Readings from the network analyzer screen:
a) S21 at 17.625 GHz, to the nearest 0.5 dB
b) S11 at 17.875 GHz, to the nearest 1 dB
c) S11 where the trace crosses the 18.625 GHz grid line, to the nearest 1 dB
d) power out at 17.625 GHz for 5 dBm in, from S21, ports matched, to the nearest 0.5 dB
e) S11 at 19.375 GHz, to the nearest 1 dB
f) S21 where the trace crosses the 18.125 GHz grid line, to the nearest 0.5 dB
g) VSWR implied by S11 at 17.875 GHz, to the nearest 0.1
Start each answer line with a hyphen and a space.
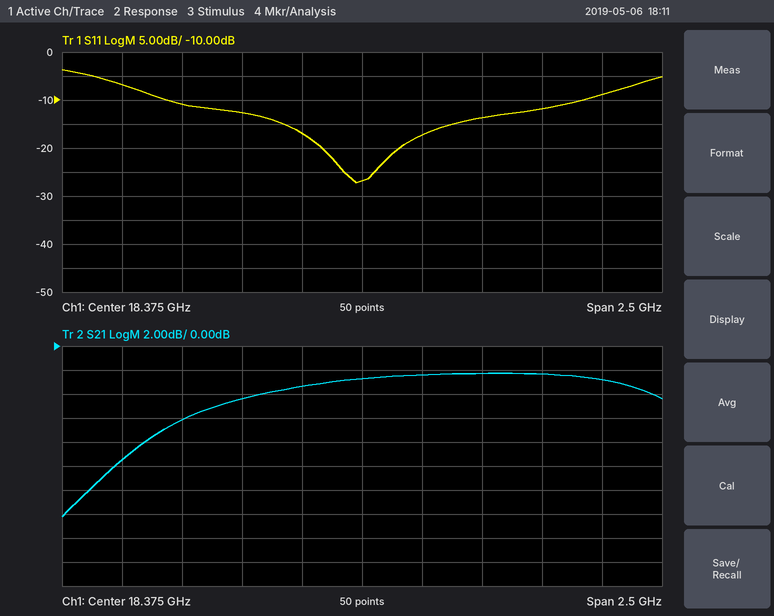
- -6.0 dB
- -13 dB
- -17 dB
- -1.0 dBm
- -9 dB
- -3.5 dB
- 1.6
